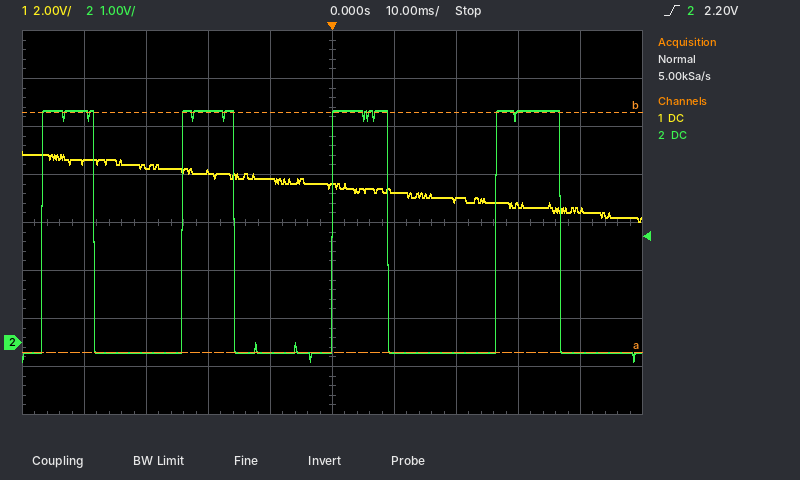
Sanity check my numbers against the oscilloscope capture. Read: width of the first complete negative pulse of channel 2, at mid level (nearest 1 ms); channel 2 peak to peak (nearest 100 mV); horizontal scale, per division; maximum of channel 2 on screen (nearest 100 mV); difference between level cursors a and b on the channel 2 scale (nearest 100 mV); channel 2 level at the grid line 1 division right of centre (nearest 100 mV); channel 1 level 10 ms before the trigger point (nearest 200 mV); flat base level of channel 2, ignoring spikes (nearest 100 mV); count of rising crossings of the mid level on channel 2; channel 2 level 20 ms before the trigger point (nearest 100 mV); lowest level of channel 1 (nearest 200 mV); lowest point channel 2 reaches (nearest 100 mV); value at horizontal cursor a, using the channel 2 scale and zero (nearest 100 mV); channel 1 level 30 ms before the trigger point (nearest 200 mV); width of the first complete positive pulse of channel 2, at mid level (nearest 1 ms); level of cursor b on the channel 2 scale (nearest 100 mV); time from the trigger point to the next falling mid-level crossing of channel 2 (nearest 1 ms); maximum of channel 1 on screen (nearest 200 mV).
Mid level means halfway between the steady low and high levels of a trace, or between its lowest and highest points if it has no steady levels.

14 ms
5.2 V
10 ms
4.8 V
5.0 V
-200 mV
6.8 V
-200 mV
4
4.8 V
5.0 V
-400 mV
-200 mV
7.4 V
8 ms
4.8 V
9 ms
8.0 V
